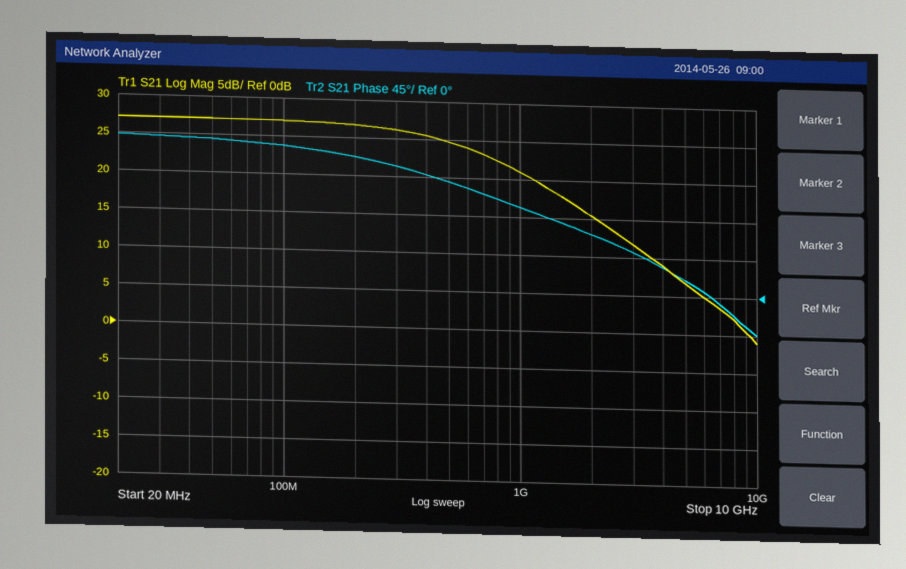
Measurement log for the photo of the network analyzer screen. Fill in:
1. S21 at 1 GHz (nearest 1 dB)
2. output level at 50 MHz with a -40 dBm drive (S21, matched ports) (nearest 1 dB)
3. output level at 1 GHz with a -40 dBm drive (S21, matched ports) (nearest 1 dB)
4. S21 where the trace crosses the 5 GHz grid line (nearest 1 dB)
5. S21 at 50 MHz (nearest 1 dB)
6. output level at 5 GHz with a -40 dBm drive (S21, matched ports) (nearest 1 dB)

21 dB
-13 dBm
-19 dBm
7 dB
27 dB
-33 dBm
